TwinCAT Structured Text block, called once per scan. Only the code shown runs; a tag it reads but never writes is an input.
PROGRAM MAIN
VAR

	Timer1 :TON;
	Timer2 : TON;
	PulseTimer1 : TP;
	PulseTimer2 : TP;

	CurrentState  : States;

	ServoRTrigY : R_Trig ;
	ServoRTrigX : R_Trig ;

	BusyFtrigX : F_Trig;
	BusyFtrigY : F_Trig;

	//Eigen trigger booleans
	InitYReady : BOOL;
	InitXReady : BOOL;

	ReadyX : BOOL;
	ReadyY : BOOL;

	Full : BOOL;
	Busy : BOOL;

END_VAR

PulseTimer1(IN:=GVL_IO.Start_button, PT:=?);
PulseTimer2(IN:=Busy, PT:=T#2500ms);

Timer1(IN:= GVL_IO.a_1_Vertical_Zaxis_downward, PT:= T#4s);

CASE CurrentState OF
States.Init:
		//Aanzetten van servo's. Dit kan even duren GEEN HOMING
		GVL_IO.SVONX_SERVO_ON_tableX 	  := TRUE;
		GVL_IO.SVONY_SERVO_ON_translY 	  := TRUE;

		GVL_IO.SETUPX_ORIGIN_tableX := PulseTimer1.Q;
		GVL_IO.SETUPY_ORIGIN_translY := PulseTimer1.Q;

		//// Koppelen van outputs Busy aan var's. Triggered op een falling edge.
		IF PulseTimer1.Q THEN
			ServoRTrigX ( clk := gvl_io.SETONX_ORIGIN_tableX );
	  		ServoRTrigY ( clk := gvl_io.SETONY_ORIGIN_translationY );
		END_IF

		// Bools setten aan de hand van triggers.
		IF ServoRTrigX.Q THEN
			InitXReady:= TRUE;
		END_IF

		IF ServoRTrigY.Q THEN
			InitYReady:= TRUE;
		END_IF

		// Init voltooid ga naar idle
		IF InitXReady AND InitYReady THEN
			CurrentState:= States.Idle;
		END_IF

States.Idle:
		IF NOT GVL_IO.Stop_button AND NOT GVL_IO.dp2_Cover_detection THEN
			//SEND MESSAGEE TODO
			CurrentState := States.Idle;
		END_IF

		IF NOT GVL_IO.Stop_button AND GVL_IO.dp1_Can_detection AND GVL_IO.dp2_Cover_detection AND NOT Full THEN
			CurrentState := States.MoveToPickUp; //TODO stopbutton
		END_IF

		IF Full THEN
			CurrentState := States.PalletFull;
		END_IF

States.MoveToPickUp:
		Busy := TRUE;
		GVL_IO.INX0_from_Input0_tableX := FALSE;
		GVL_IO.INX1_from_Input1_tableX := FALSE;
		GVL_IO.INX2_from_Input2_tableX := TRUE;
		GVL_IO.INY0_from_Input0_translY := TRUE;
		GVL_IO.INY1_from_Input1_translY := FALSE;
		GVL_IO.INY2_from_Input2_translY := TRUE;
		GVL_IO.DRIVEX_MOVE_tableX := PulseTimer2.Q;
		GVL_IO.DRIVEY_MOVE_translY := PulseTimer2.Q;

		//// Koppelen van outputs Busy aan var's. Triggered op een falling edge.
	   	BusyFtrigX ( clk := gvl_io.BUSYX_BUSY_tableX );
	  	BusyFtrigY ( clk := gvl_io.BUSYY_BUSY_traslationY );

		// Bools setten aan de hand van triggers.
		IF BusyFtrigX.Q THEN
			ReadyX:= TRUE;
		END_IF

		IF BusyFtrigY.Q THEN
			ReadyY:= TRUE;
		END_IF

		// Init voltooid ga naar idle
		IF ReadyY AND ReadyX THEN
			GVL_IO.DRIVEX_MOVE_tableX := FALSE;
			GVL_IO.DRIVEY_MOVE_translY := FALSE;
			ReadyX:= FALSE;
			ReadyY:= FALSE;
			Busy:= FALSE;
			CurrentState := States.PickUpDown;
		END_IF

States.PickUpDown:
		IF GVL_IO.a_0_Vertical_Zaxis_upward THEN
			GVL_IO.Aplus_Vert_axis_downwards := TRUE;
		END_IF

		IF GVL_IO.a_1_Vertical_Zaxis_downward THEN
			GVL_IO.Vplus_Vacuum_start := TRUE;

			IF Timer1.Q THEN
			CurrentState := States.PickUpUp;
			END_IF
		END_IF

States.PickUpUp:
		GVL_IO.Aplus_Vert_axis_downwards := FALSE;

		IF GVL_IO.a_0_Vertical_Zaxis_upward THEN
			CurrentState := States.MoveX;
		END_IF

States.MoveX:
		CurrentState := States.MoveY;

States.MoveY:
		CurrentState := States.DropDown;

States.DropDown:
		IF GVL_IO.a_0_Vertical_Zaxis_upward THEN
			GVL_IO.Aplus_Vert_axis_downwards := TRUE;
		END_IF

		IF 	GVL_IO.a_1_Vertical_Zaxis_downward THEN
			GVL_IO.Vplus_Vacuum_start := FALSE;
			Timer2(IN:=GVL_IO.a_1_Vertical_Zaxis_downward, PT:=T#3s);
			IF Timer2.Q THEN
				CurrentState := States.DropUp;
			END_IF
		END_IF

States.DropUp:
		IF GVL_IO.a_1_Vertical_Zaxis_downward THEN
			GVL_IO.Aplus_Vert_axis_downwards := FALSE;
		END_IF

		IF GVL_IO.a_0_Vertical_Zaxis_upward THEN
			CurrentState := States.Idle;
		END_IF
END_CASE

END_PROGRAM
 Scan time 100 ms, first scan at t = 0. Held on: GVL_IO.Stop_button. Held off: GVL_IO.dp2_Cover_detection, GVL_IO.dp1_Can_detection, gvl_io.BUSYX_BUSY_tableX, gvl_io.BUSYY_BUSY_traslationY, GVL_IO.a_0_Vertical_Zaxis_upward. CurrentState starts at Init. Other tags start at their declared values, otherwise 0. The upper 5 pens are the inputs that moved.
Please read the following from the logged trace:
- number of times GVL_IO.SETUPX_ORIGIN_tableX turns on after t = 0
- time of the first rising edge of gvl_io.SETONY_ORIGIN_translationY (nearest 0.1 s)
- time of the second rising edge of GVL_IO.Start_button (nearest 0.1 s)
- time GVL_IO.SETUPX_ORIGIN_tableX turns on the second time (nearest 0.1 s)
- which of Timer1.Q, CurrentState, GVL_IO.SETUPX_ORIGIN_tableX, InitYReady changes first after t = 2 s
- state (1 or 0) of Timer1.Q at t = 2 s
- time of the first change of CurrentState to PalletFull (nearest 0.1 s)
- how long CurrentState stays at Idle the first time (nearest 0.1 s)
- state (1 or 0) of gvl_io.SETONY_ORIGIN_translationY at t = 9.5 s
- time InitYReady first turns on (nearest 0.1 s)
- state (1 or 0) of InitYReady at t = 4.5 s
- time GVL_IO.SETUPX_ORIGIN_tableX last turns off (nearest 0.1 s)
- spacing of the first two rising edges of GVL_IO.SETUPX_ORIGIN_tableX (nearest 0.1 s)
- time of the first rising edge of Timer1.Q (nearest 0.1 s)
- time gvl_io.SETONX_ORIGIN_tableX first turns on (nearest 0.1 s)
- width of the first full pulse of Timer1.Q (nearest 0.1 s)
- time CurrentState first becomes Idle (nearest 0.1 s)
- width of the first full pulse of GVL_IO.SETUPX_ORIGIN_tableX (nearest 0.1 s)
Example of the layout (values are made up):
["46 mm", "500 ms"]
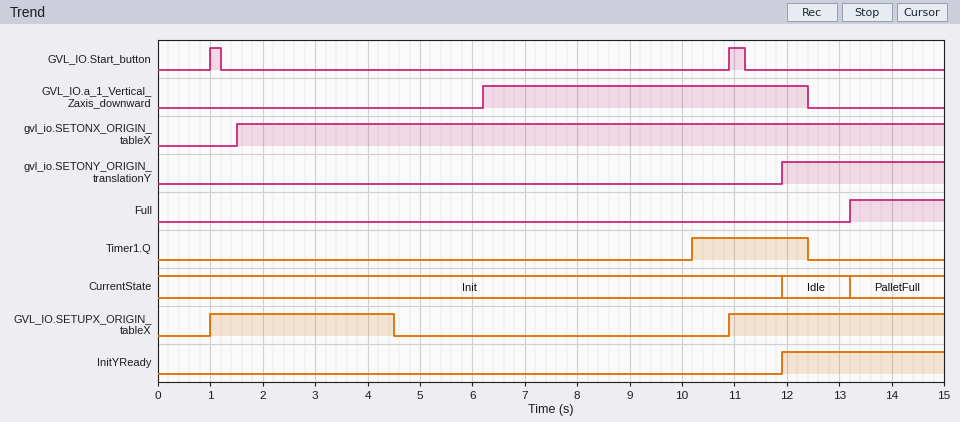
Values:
["2", "11.9 s", "10.9 s", "10.9 s", "GVL_IO.SETUPX_ORIGIN_tableX", "0", "13.2 s", "1.3 s", "0", "11.9 s", "0", "4.5 s", "9.9 s", "10.2 s", "1.5 s", "2.2 s", "11.9 s", "3.5 s"]
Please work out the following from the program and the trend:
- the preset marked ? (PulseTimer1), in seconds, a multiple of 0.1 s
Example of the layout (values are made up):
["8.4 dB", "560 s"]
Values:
["3.5 s"]
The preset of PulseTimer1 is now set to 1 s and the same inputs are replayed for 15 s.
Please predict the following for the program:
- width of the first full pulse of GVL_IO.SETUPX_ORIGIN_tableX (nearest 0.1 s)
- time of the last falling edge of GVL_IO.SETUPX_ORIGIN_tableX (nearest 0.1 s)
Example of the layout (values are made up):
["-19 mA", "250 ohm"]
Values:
["1.0 s", "11.9 s"]
